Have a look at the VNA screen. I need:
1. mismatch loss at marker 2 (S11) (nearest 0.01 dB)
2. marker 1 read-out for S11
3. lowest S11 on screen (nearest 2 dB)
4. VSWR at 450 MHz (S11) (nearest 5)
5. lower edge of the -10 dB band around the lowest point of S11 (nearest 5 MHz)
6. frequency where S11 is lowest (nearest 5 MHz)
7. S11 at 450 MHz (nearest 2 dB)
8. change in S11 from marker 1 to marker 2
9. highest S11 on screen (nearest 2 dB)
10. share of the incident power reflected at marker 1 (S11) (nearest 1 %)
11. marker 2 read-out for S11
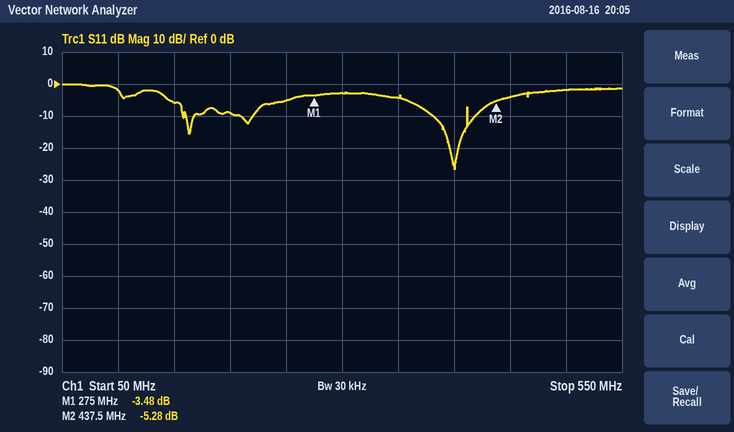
1.53 dB
-3.48 dB
-26 dB
5
380 MHz
400 MHz
-4 dB
-1.80 dB
0 dB
45 %
-5.28 dB
